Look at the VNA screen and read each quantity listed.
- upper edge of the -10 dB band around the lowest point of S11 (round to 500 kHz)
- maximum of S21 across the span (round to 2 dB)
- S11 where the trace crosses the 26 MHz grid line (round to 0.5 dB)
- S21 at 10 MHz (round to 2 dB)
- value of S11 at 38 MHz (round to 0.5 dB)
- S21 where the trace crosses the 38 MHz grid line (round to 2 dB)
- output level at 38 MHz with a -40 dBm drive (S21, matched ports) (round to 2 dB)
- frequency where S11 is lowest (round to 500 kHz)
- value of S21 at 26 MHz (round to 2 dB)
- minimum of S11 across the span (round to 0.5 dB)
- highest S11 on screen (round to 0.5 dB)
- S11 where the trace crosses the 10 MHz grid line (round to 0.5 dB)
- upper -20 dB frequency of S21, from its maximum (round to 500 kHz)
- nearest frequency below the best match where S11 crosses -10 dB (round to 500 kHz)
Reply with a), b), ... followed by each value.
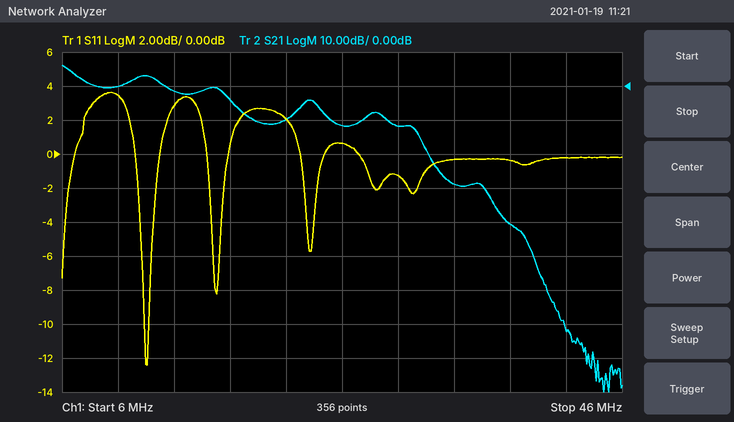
a) 12.0 MHz
b) 6 dB
c) 0.5 dB
d) 0 dB
e) -0.5 dB
f) -40 dB
g) -80 dBm
h) 12.0 MHz
i) -12 dB
j) -12.5 dB
k) 3.5 dB
l) 3.5 dB
m) 31.5 MHz
n) 12.0 MHz
